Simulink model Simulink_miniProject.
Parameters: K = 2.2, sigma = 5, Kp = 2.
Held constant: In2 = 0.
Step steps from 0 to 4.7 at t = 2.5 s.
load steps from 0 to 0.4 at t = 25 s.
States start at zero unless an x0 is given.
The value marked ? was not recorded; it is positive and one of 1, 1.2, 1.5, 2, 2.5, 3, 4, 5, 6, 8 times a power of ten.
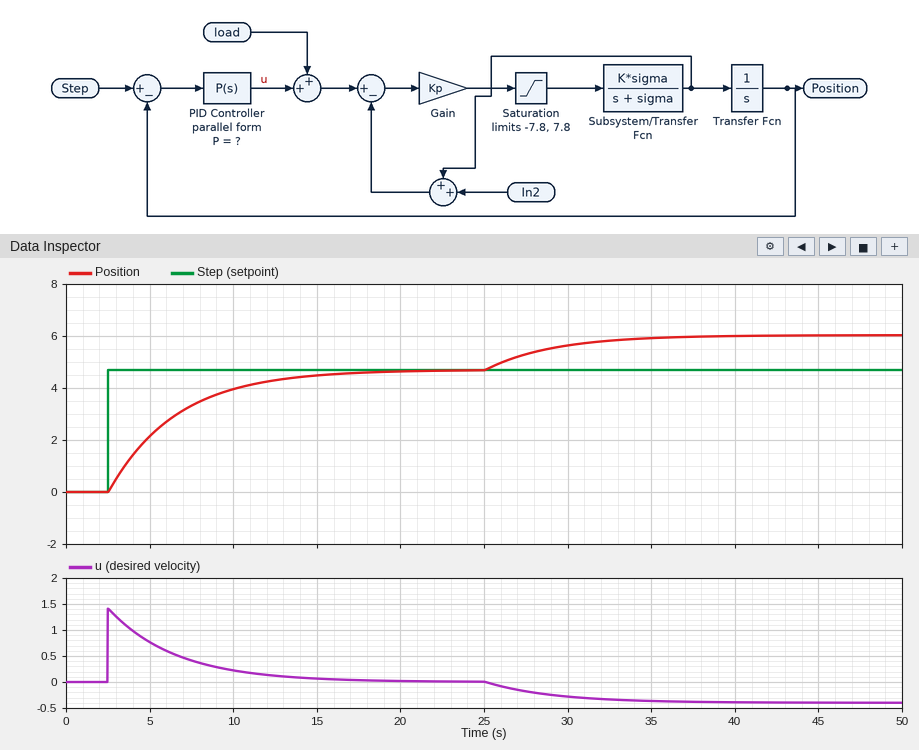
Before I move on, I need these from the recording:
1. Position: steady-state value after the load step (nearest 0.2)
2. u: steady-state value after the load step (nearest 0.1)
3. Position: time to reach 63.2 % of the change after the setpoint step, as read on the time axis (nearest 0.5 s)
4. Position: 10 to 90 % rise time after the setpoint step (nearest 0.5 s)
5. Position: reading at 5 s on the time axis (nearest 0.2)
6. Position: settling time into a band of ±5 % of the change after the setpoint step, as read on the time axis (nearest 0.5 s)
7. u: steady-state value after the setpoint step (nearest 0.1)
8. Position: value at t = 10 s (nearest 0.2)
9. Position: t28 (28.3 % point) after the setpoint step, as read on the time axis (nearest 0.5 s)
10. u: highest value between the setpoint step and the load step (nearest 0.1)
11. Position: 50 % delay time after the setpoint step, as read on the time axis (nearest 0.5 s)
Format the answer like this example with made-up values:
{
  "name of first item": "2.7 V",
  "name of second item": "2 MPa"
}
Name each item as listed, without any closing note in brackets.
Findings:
{
  "Position: steady-state value after the load step": "6.0",
  "u: steady-state value after the load step": "-0.4",
  "Position: time to reach 63.2 % of the change after the setpoint step, as read on the time axis": "6.5 s",
  "Position: 10 to 90 % rise time after the setpoint step": "9.0 s",
  "Position: reading at 5 s on the time axis": "2.2",
  "Position: settling time into a band of ±5 % of the change after the setpoint step, as read on the time axis": "14.5 s",
  "u: steady-state value after the setpoint step": "0.0",
  "Position: value at t = 10 s": "4.0",
  "Position: t28 (28.3 % point) after the setpoint step, as read on the time axis": "4.0 s",
  "u: highest value between the setpoint step and the load step": "1.4",
  "Position: 50 % delay time after the setpoint step, as read on the time axis": "5.5 s"
}
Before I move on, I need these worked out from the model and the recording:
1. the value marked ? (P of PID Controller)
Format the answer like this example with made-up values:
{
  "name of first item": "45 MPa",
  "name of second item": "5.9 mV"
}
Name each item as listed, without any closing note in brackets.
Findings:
{
  "the value marked ?": "0.3"
}
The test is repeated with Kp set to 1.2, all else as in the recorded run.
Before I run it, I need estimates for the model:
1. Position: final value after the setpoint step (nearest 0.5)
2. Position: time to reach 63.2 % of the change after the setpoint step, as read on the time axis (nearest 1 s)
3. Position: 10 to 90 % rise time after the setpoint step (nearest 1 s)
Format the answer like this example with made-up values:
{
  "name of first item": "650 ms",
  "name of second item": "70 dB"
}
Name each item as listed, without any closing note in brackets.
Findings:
{
  "Position: final value after the setpoint step": "4.5",
  "Position: time to reach 63.2 % of the change after the setpoint step, as read on the time axis": "7 s",
  "Position: 10 to 90 % rise time after the setpoint step": "10 s"
}
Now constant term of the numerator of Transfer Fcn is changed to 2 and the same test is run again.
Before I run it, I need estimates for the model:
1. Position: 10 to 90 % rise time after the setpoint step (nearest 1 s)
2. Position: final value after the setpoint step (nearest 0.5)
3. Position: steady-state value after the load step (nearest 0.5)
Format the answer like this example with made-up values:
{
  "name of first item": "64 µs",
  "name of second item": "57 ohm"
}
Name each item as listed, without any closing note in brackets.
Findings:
{
  "Position: 10 to 90 % rise time after the setpoint step": "4 s",
  "Position: final value after the setpoint step": "4.5",
  "Position: steady-state value after the load step": "6.0"
}
